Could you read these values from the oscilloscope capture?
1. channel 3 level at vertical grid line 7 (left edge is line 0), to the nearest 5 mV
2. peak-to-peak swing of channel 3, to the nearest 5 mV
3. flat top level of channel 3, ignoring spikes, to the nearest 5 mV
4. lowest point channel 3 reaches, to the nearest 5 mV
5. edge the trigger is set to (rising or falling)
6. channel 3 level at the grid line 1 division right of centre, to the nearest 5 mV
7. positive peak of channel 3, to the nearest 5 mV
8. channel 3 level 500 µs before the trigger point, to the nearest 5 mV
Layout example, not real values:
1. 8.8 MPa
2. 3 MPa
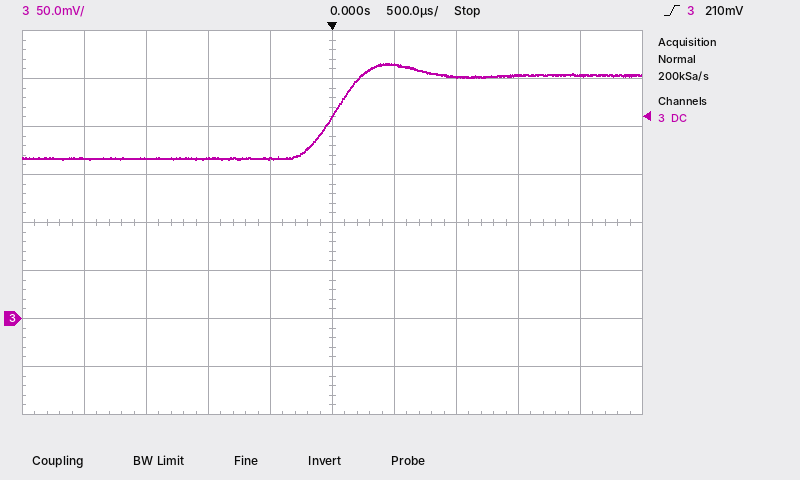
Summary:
1. 250 mV
2. 100 mV
3. 255 mV
4. 165 mV
5. rising
6. 265 mV
7. 265 mV
8. 165 mV
